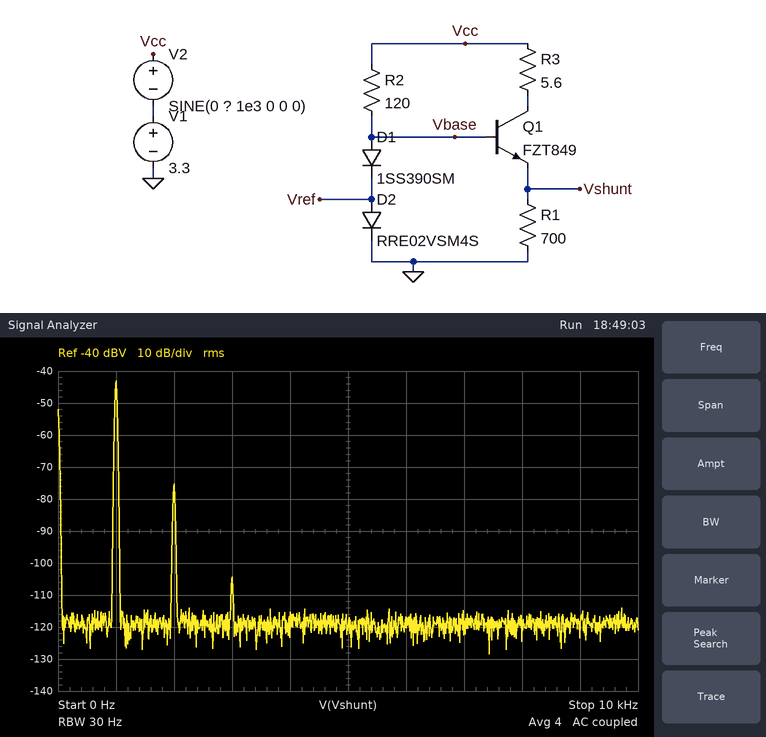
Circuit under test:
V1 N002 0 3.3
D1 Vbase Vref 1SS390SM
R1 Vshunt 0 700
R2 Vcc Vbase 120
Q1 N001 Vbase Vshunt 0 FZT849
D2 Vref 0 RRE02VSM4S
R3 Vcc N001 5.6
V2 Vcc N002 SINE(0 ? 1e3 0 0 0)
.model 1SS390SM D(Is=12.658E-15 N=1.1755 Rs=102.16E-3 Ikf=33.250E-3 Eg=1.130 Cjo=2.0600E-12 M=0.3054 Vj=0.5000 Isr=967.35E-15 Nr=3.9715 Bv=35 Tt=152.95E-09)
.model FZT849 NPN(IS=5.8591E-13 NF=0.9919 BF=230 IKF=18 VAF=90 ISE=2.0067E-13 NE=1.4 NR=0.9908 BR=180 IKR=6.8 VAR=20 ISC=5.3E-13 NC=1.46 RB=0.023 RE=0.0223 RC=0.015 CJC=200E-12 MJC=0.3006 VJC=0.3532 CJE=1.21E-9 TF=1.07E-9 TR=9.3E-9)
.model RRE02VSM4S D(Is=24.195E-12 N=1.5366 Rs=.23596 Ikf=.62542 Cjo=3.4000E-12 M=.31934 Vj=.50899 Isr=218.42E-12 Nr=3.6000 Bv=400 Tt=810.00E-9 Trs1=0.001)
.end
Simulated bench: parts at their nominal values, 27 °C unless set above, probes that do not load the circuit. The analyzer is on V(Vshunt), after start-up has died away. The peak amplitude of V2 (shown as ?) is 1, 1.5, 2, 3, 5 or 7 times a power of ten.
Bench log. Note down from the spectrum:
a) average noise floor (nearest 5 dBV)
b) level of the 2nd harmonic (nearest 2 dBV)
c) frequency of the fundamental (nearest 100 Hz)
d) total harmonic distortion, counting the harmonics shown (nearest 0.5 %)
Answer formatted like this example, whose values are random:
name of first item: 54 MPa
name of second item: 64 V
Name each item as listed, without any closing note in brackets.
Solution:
average noise floor: -120 dBV
level of the 2nd harmonic: -76 dBV
frequency of the fundamental: 1.0 kHz
total harmonic distortion, counting the harmonics shown: 2.5 %
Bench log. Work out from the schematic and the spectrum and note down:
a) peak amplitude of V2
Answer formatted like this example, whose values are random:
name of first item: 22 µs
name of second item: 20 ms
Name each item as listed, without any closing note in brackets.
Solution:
peak amplitude of V2: 200 mV
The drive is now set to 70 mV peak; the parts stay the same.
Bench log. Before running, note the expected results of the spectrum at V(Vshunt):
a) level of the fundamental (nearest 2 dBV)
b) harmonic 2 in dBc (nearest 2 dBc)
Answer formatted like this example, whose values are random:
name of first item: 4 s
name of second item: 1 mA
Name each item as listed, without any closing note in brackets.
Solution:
level of the fundamental: -52 dBV
harmonic 2 in dBc: -42 dBc
